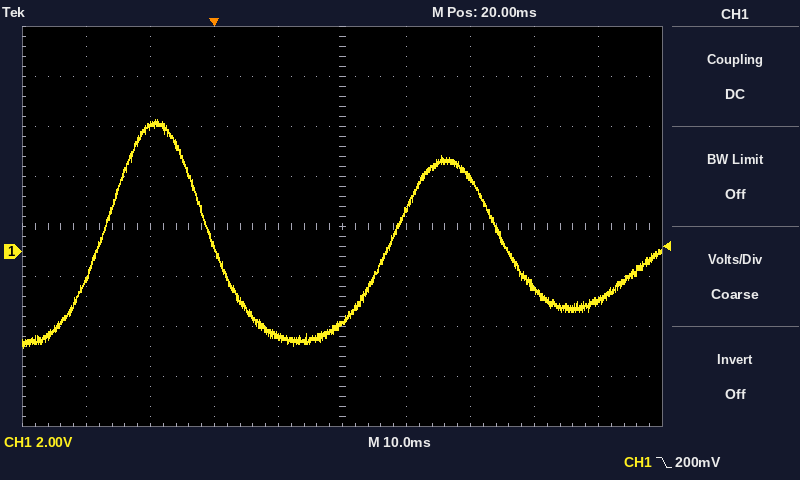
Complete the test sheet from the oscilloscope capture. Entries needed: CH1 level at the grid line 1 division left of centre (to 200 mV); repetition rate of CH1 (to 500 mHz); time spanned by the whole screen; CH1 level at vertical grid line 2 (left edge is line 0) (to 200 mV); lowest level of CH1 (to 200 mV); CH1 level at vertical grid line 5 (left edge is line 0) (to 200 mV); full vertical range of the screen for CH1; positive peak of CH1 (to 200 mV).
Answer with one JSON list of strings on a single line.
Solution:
["-3.4 V", "22.0 Hz", "100 ms", "5.0 V", "-3.8 V", "-2.8 V", "16 V", "5.2 V"]
